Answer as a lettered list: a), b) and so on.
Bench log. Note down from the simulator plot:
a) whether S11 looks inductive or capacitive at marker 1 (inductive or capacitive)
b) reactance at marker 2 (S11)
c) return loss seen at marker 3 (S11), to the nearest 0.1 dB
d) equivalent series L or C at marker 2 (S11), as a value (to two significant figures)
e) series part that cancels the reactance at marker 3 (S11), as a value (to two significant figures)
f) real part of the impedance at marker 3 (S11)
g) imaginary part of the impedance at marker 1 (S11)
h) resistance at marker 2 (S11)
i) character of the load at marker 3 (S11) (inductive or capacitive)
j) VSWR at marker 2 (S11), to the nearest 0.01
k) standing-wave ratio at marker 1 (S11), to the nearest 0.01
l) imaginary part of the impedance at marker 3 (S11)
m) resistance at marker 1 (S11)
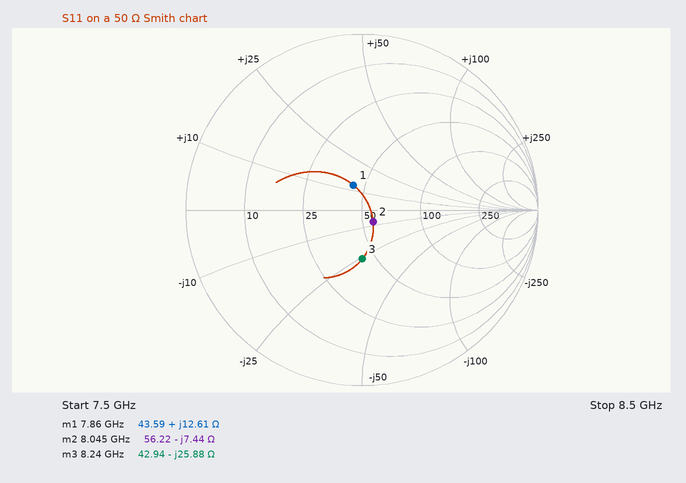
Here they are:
a) inductive
b) -7.44 Ω
c) 11.1 dB
d) 2.7 pF
e) 500 pH
f) 42.94 Ω
g) +12.61 Ω
h) 56.22 Ω
i) capacitive
j) 1.20
k) 1.35
l) -25.88 Ω
m) 43.59 Ω
